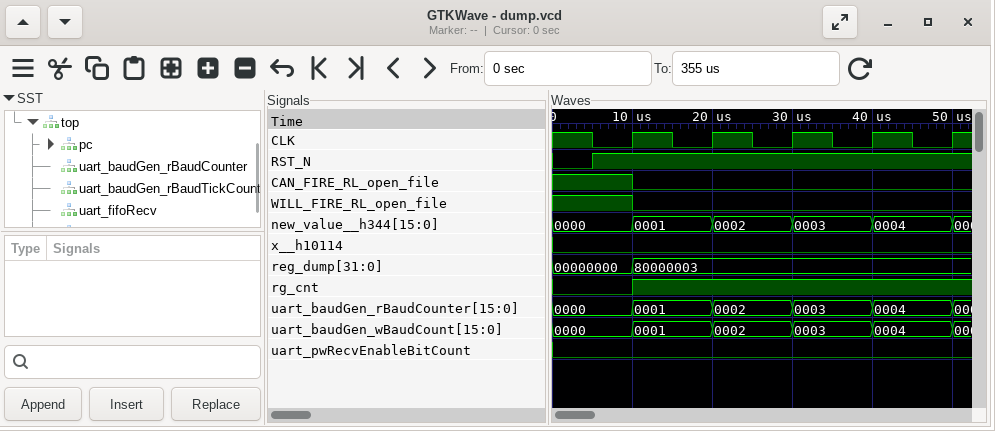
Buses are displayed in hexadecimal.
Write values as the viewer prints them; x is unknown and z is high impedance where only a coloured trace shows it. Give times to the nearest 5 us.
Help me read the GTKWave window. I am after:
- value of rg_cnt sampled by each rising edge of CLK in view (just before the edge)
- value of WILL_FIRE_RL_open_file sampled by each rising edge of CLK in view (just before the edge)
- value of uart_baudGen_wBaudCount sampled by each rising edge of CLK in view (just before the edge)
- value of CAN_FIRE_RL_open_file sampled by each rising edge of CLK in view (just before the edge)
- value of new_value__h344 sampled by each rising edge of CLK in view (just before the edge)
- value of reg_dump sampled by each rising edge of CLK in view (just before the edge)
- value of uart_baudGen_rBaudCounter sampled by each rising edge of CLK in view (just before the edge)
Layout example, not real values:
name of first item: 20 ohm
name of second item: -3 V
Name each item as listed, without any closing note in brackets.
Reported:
value of rg_cnt sampled by each rising edge of CLK in view: 0 1 1 1 1
value of WILL_FIRE_RL_open_file sampled by each rising edge of CLK in view: 1 0 0 0 0
value of uart_baudGen_wBaudCount sampled by each rising edge of CLK in view: 0000, 0001, 0002, 0003, 0004
value of CAN_FIRE_RL_open_file sampled by each rising edge of CLK in view: 1 0 0 0 0
value of new_value__h344 sampled by each rising edge of CLK in view: 0000, 0001, 0002, 0003, 0004
value of reg_dump sampled by each rising edge of CLK in view: 00000000, 80000003, 80000003, 80000003, 80000003
value of uart_baudGen_rBaudCounter sampled by each rising edge of CLK in view: 0000, 0001, 0002, 0003, 0004
